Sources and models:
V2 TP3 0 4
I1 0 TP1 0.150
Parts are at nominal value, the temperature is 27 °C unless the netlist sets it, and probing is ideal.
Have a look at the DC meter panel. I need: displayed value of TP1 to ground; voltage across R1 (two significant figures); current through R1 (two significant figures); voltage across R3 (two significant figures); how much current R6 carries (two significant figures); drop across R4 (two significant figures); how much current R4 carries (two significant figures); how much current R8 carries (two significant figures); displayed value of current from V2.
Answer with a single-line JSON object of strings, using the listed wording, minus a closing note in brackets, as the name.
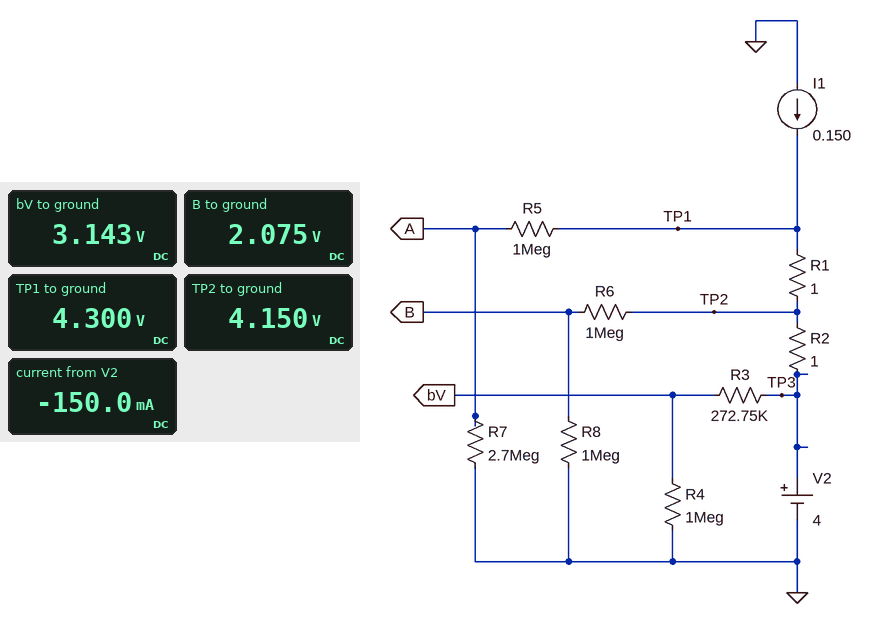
{"displayed value of TP1 to ground": "4.300 V", "voltage across R1": "150 mV", "current through R1": "150 mA", "voltage across R3": "860 mV", "how much current R6 carries": "2.1 µA", "drop across R4": "3.1 V", "how much current R4 carries": "3.1 µA", "how much current R8 carries": "2.1 µA", "displayed value of current from V2": "-150.0 mA"}
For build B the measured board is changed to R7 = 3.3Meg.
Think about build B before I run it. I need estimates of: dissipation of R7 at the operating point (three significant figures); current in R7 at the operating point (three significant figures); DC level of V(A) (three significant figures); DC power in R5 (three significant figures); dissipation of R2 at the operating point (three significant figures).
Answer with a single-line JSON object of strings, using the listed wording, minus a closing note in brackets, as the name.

{"dissipation of R7 at the operating point": "3.30 µW", "current in R7 at the operating point": "1.00 µA", "DC level of V(A)": "3.30 V", "DC power in R5": "1.00 µW", "dissipation of R2 at the operating point": "22.5 mW"}
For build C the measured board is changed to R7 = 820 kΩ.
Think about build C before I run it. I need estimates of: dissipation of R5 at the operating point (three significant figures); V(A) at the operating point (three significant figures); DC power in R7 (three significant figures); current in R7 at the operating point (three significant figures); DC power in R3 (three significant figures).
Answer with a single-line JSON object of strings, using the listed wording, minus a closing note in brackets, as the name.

{"dissipation of R5 at the operating point": "5.58 µW", "V(A) at the operating point": "1.94 V", "DC power in R7": "4.58 µW", "current in R7 at the operating point": "2.36 µA", "DC power in R3": "2.69 µW"}
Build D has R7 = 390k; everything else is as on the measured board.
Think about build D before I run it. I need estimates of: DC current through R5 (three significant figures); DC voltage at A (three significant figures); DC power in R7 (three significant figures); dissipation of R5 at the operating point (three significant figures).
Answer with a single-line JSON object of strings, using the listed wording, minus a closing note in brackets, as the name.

{"DC current through R5": "3.09 µA", "DC voltage at A": "1.21 V", "DC power in R7": "3.73 µW", "dissipation of R5 at the operating point": "9.57 µW"}
